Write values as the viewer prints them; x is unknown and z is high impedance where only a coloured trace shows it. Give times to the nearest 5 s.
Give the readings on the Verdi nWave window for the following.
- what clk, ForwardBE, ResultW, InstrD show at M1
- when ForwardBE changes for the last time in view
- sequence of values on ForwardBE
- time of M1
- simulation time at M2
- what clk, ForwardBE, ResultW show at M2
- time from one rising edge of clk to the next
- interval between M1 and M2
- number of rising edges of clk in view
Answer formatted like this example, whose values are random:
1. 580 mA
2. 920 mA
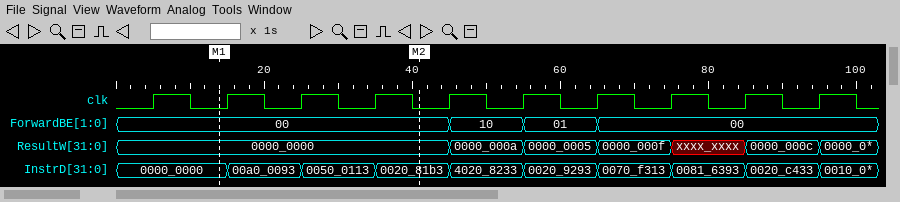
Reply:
1. clk=0, ForwardBE=00, ResultW=0000_0000, InstrD=0000_0000
2. 65 s
3. 00, 10, 01, 00
4. 15 s
5. 40 s
6. clk=0, ForwardBE=00, ResultW=0000_0000
7. 10 s
8. 25 s
9. 10
